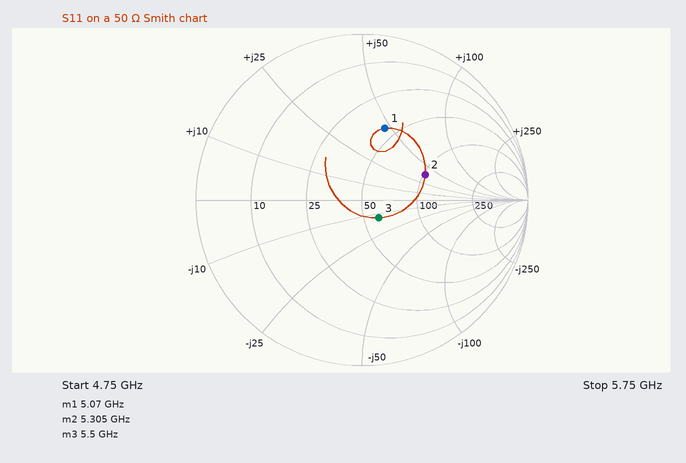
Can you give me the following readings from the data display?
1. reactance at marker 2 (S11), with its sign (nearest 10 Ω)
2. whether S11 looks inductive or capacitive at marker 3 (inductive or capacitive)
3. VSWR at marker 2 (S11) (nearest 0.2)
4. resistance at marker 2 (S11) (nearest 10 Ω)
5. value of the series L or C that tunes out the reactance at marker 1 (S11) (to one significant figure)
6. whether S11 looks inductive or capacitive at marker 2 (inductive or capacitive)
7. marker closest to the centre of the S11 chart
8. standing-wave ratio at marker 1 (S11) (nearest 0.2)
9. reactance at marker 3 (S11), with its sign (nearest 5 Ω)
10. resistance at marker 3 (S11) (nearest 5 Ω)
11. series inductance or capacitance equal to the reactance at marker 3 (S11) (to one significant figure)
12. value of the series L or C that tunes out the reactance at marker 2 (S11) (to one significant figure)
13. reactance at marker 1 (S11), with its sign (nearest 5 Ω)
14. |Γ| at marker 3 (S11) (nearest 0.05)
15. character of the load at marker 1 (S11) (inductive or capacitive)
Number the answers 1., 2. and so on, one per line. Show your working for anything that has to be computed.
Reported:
1. +40 Ω
2. capacitive
3. 2.4
4. 100 Ω
5. C = 1/(2π × 5.07 GHz × 45 Ω) ≈ 698 fF, so 700 fF to one significant figure
6. inductive
7. marker 3
8. 2.6
9. -15 Ω
10. 60 Ω
11. C = 1/(2π × 5.5 GHz × 15 Ω) ≈ 2 pF
12. C = 1/(2π × 5.305 GHz × 40 Ω) ≈ 750 fF, so 800 fF to one significant figure
13. +45 Ω
14. 0.15
15. inductive
